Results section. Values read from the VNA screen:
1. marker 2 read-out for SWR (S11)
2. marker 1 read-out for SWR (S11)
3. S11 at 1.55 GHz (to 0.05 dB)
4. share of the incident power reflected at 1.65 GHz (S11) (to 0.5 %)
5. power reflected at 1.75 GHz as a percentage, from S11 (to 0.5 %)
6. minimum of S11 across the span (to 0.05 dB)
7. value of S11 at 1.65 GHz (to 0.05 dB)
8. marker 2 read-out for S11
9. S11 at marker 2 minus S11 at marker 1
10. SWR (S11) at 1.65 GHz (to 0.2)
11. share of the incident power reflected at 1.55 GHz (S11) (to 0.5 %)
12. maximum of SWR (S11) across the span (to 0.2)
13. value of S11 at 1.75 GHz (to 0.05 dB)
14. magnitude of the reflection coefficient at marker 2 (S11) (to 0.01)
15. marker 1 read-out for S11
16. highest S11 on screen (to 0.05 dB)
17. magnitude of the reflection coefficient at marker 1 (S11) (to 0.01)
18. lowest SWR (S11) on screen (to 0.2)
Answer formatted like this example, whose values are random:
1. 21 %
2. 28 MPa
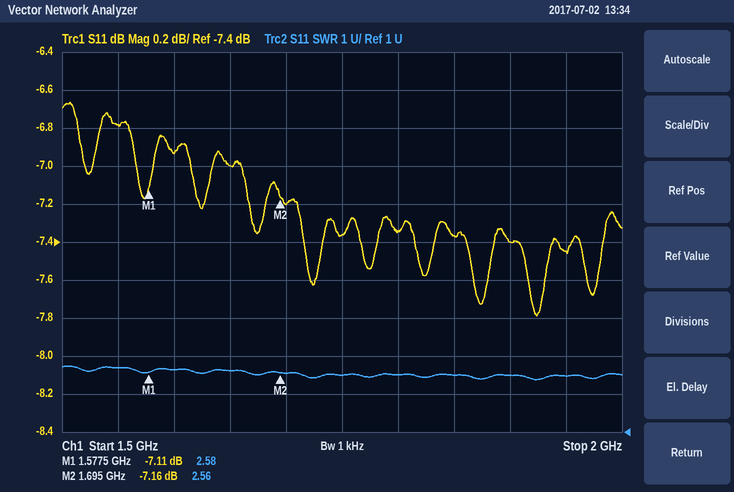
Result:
1. 2.56
2. 2.58
3. -6.80 dB
4. 20.0 %
5. 18.5 %
6. -7.80 dB
7. -7.00 dB
8. -7.16 dB
9. -0.05 dB
10. 2.6
11. 21.0 %
12. 2.8
13. -7.35 dB
14. 0.44
15. -7.11 dB
16. -6.65 dB
17. 0.44
18. 2.4
